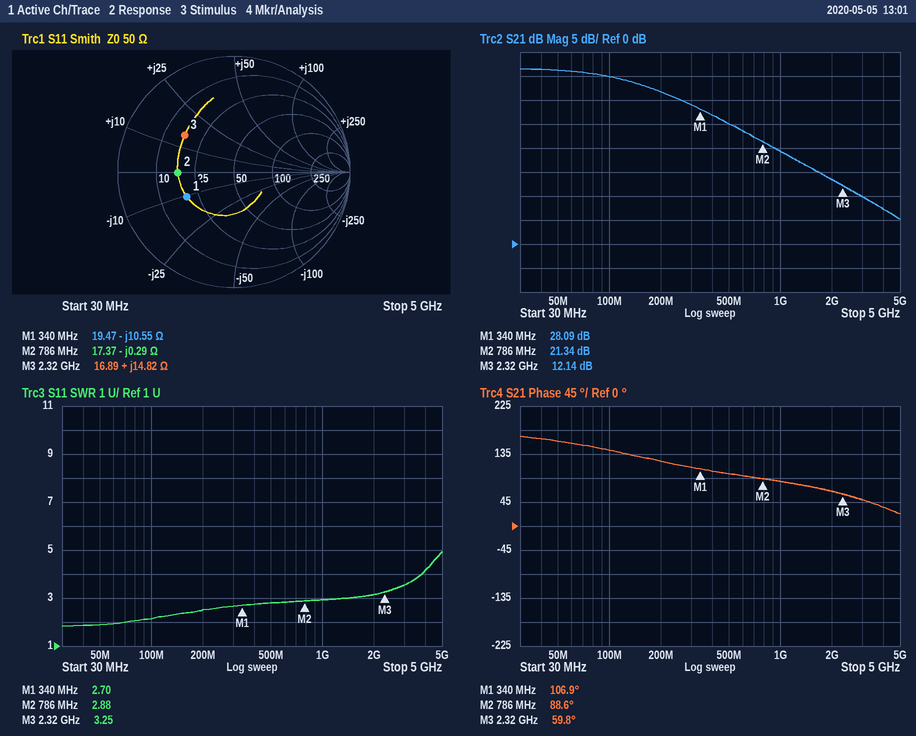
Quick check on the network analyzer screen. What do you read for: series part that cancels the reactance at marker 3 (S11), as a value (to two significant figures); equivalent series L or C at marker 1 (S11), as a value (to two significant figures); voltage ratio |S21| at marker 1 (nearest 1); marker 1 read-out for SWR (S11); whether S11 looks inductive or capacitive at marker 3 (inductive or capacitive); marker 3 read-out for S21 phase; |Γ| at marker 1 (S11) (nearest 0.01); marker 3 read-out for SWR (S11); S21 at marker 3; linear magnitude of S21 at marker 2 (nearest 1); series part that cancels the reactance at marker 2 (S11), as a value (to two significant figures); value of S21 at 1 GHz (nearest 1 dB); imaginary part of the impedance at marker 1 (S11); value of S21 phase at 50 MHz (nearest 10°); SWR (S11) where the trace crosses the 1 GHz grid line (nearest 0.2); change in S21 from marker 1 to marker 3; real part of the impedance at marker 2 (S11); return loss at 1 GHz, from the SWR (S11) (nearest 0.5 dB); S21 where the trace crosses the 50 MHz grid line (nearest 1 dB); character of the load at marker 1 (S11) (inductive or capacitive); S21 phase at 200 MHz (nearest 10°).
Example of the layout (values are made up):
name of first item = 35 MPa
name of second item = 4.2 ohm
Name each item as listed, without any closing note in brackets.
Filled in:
series part that cancels the reactance at marker 3 (S11), as a value = 4.6 pF
equivalent series L or C at marker 1 (S11), as a value = 44 pF
voltage ratio |S21| at marker 1 = 25
marker 1 read-out for SWR = 2.70
whether S11 looks inductive or capacitive at marker 3 = inductive
marker 3 read-out for S21 phase = 59.8°
|Γ| at marker 1 (S11) = 0.46
marker 3 read-out for SWR = 3.25
S21 at marker 3 = 12.14 dB
linear magnitude of S21 at marker 2 = 12
series part that cancels the reactance at marker 2 (S11), as a value = 59 pH
value of S21 at 1 GHz = 19 dB
imaginary part of the impedance at marker 1 = -10.55 Ω
value of S21 phase at 50 MHz = 160°
SWR (S11) where the trace crosses the 1 GHz grid line = 3.0
change in S21 from marker 1 to marker 3 = -15.95 dB
real part of the impedance at marker 2 = 17.37 Ω
return loss at 1 GHz, from the SWR (S11) = 6.0 dB
S21 where the trace crosses the 50 MHz grid line = 36 dB
character of the load at marker 1 (S11) = capacitive
S21 phase at 200 MHz = 120°
